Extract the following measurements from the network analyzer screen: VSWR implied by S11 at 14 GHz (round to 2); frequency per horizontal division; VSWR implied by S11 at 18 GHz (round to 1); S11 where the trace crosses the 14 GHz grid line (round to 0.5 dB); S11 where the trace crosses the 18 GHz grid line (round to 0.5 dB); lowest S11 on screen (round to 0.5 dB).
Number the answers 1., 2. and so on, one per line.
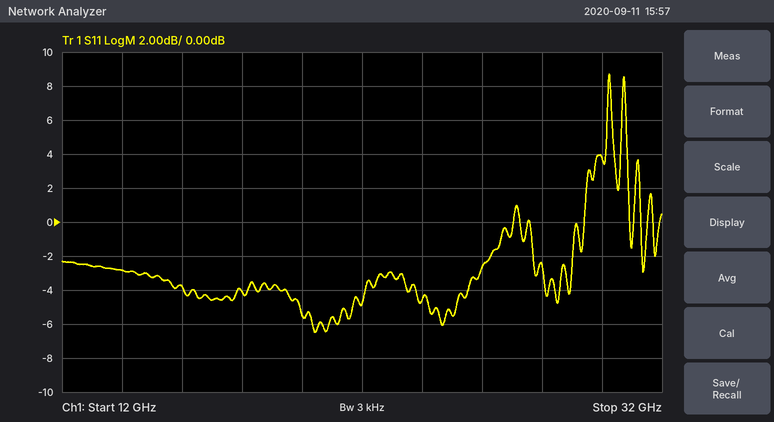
1. 6
2. 2 GHz
3. 4
4. -3.0 dB
5. -4.0 dB
6. -6.5 dB
